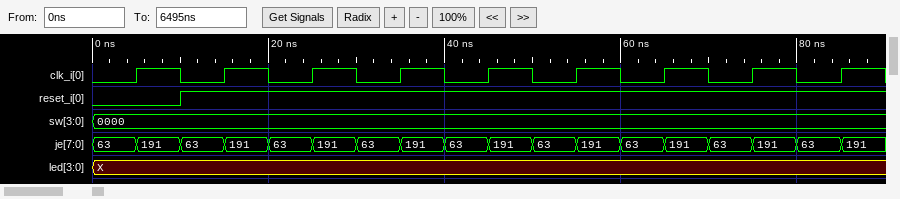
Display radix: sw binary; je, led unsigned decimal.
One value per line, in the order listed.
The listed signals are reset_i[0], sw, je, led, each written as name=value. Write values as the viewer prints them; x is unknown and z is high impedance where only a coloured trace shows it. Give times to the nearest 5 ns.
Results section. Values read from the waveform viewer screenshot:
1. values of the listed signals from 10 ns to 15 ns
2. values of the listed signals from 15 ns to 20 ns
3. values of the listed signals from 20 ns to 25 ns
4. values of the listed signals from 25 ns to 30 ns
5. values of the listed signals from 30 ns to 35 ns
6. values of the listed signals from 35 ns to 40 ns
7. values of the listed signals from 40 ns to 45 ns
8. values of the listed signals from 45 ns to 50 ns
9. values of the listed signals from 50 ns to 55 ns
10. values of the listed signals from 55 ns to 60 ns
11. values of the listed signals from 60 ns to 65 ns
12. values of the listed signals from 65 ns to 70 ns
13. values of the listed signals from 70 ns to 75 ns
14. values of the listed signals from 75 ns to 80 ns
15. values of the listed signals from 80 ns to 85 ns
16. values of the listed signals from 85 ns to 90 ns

reset_i[0]=1, sw=0000, je=63, led=X
reset_i[0]=1, sw=0000, je=191, led=X
reset_i[0]=1, sw=0000, je=63, led=X
reset_i[0]=1, sw=0000, je=191, led=X
reset_i[0]=1, sw=0000, je=63, led=X
reset_i[0]=1, sw=0000, je=191, led=X
reset_i[0]=1, sw=0000, je=63, led=X
reset_i[0]=1, sw=0000, je=191, led=X
reset_i[0]=1, sw=0000, je=63, led=X
reset_i[0]=1, sw=0000, je=191, led=X
reset_i[0]=1, sw=0000, je=63, led=X
reset_i[0]=1, sw=0000, je=191, led=X
reset_i[0]=1, sw=0000, je=63, led=X
reset_i[0]=1, sw=0000, je=191, led=X
reset_i[0]=1, sw=0000, je=63, led=X
reset_i[0]=1, sw=0000, je=191, led=X
